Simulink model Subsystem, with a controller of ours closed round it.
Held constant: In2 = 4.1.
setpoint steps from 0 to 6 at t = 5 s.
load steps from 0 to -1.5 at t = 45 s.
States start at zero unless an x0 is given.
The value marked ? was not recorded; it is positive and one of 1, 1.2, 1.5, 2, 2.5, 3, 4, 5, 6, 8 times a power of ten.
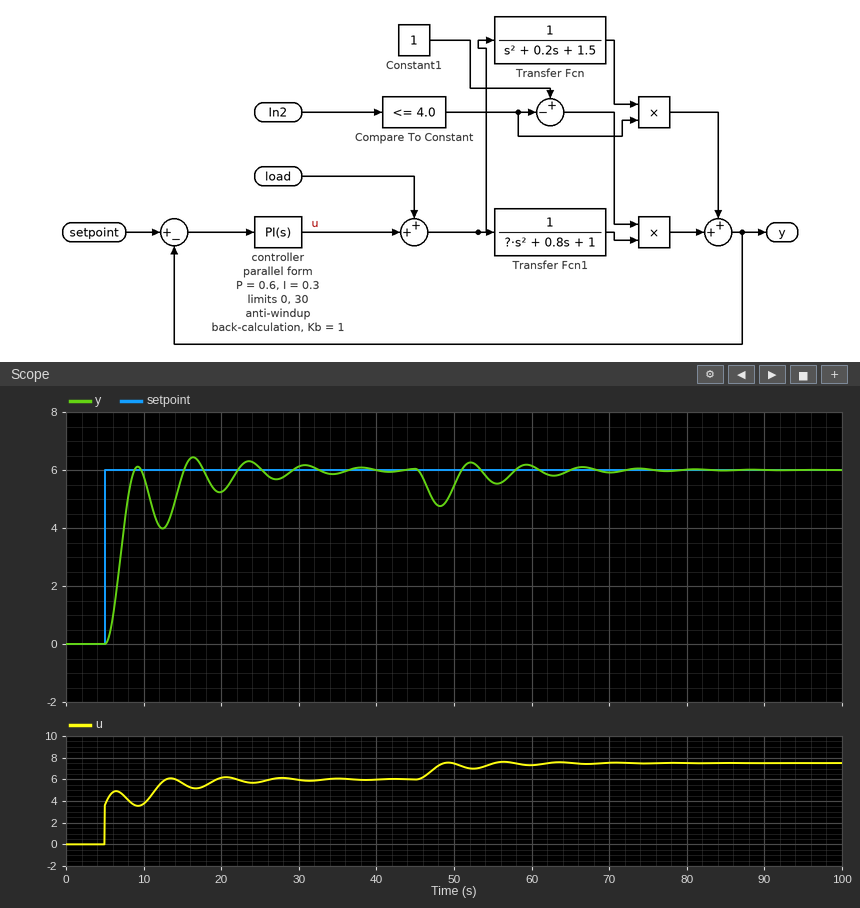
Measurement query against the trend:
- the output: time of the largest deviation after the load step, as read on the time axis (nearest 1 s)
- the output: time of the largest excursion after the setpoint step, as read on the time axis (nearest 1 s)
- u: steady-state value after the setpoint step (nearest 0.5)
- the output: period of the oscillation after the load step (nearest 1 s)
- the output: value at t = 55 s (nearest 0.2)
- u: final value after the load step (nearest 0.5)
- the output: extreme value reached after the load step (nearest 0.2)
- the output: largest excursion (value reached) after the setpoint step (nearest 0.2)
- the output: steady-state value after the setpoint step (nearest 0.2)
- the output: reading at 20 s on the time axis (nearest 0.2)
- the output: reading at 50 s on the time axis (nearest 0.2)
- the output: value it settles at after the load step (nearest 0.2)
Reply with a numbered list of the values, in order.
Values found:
1. 48 s
2. 16 s
3. 6.0
4. 7 s
5. 5.6
6. 7.5
7. 4.8
8. 6.4
9. 6.0
10. 5.2
11. 5.4
12. 6.0
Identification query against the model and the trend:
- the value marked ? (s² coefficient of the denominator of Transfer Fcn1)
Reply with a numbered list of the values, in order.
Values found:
1. 2
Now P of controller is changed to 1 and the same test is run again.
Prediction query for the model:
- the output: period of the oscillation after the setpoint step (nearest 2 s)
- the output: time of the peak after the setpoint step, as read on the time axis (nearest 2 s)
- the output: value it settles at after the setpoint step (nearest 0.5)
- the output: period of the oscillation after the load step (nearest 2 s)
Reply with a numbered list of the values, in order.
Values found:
1. 6 s
2. 8 s
3. 6.0
4. 6 s
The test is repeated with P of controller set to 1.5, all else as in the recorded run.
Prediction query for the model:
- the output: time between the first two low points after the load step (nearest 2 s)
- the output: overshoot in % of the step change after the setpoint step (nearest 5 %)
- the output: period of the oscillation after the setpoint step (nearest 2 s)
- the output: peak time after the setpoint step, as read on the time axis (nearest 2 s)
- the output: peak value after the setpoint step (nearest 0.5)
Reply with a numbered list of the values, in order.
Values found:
1. 6 s
2. 15 %
3. 6 s
4. 8 s
5. 7.0
